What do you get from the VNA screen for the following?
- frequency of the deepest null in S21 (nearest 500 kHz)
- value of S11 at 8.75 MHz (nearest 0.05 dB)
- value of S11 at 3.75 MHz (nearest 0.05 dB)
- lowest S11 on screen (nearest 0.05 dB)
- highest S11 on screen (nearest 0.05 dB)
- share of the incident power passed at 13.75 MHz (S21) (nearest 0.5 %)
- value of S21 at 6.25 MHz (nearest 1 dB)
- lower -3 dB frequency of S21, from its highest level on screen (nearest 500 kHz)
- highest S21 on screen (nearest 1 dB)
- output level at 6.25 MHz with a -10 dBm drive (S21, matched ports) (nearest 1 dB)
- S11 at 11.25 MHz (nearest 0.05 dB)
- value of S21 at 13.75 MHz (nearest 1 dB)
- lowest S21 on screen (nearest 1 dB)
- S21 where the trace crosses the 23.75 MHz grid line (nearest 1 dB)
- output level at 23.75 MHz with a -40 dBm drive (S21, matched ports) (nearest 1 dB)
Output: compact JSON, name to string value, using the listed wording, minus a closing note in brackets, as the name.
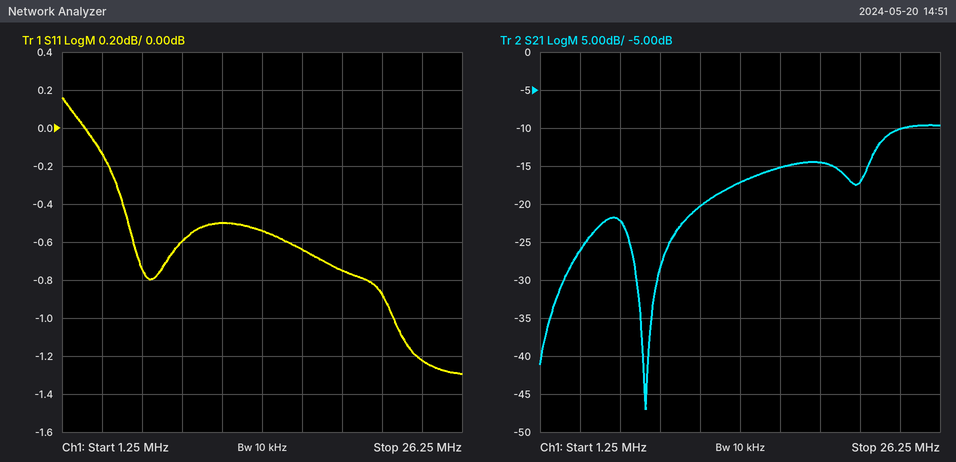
{"frequency of the deepest null in S21": "8.0 MHz", "value of S11 at 8.75 MHz": "-0.60 dB", "value of S11 at 3.75 MHz": "-0.15 dB", "lowest S11 on screen": "-1.30 dB", "highest S11 on screen": "0.15 dB", "share of the incident power passed at 13.75 MHz (S21)": "2.0 %", "value of S21 at 6.25 MHz": "-22 dB", "lower -3 dB frequency of S21, from its highest level on screen": "22.5 MHz", "highest S21 on screen": "-10 dB", "output level at 6.25 MHz with a -10 dBm drive (S21, matched ports)": "-32 dBm", "S11 at 11.25 MHz": "-0.50 dB", "value of S21 at 13.75 MHz": "-17 dB", "lowest S21 on screen": "-47 dB", "S21 where the trace crosses the 23.75 MHz grid line": "-10 dB", "output level at 23.75 MHz with a -40 dBm drive (S21, matched ports)": "-50 dBm"}
